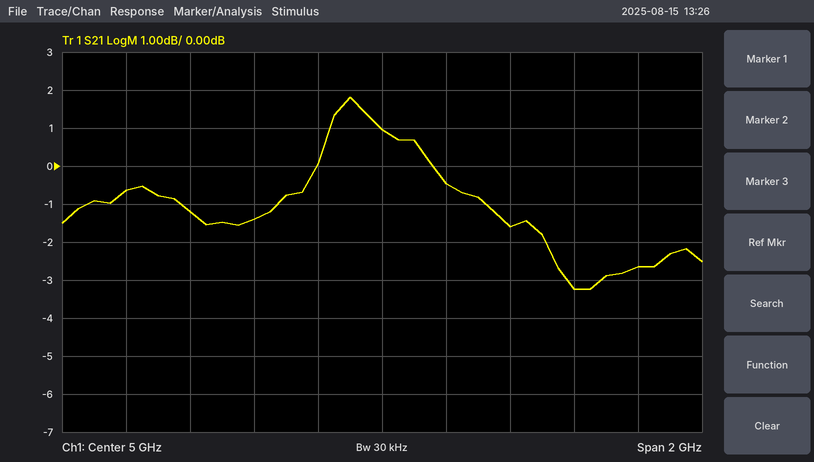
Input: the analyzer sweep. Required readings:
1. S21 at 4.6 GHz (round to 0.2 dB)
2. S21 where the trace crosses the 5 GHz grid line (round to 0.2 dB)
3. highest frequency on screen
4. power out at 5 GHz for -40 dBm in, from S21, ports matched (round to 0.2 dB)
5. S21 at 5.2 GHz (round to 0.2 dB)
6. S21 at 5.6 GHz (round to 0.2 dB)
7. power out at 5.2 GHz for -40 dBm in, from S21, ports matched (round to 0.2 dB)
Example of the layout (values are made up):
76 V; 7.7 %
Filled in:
-1.4 dB; 1.0 dB; 6 GHz; -39.0 dBm; -0.4 dB; -3.2 dB; -40.4 dBm
